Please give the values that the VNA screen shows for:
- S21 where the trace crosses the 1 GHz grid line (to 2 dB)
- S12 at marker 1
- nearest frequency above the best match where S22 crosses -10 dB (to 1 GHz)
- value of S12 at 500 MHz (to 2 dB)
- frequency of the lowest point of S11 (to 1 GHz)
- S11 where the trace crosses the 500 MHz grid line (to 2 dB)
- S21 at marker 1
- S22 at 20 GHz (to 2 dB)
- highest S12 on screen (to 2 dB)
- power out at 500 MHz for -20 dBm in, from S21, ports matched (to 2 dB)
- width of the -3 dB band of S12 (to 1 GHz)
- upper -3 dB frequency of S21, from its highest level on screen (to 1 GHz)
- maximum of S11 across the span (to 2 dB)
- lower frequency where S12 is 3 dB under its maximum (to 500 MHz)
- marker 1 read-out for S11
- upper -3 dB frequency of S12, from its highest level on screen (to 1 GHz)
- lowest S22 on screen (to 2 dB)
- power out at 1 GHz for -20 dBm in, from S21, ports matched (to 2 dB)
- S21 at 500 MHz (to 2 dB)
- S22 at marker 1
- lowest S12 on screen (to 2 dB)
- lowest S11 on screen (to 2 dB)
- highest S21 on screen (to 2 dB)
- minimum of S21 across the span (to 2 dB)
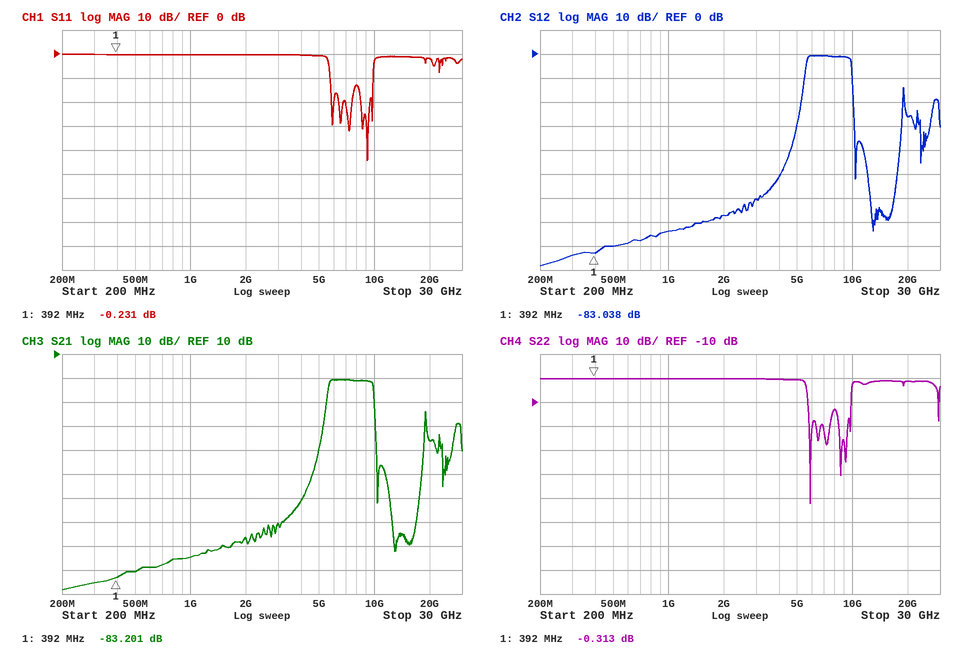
-74 dB
-83.038 dB
10 GHz
-80 dB
9 GHz
0 dB
-83.201 dB
-2 dB
0 dB
-100 dBm
4 GHz
10 GHz
0 dB
5.5 GHz
-0.231 dB
10 GHz
-52 dB
-94 dBm
-80 dB
-0.313 dB
-88 dB
-44 dB
0 dB
-88 dB
